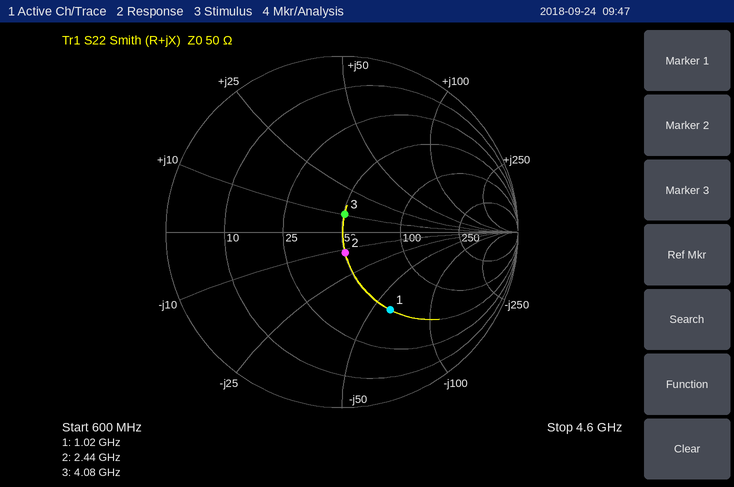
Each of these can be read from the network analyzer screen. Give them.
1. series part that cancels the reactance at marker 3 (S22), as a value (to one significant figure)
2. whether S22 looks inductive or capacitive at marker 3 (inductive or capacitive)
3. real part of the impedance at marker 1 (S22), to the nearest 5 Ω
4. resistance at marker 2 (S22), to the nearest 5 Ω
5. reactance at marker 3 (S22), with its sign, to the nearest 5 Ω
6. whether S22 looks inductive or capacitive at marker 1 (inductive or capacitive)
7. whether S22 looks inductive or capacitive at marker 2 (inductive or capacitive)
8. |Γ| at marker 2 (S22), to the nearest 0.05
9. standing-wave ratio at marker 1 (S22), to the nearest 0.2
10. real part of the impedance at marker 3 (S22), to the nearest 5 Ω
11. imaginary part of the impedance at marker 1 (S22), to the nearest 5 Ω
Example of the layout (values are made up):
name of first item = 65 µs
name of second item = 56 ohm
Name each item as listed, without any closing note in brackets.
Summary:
series part that cancels the reactance at marker 3 (S22), as a value = 4 pF
whether S22 looks inductive or capacitive at marker 3 = inductive
real part of the impedance at marker 1 (S22), to the nearest 5 Ω = 50 Ω
resistance at marker 2 (S22), to the nearest 5 Ω = 50 Ω
reactance at marker 3 (S22), with its sign, to the nearest 5 Ω = +10 Ω
whether S22 looks inductive or capacitive at marker 1 = capacitive
whether S22 looks inductive or capacitive at marker 2 = capacitive
|Γ| at marker 2 (S22), to the nearest 0.05 = 0.10
standing-wave ratio at marker 1 (S22), to the nearest 0.2 = 3.2
real part of the impedance at marker 3 (S22), to the nearest 5 Ω = 50 Ω
imaginary part of the impedance at marker 1 (S22), to the nearest 5 Ω = -60 Ω
